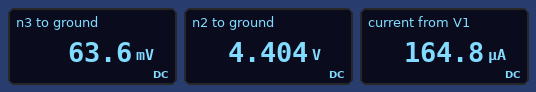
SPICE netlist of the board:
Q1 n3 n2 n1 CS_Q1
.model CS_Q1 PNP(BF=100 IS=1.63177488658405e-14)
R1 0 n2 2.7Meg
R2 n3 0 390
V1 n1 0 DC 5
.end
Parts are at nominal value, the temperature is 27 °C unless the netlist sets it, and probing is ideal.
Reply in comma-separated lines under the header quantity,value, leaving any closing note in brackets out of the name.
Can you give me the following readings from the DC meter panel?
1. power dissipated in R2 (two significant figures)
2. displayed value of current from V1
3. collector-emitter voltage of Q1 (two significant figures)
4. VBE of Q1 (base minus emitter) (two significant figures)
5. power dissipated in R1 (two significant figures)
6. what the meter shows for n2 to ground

quantity,value
power dissipated in R2,10 µW
displayed value of current from V1,164.8 µA
collector-emitter voltage of Q1,-4.9 V
VBE of Q1 (base minus emitter),-600 mV
power dissipated in R1,7.2 µW
what the meter shows for n2 to ground,4.404 V
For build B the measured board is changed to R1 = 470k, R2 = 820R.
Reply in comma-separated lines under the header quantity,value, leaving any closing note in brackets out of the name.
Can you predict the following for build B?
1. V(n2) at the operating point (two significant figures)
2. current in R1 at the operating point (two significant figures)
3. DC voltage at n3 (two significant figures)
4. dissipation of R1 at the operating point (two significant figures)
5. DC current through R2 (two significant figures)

quantity,value
V(n2) at the operating point,4.4 V
current in R1 at the operating point,9.3 µA
DC voltage at n3,760 mV
dissipation of R1 at the operating point,40 µW
DC current through R2,930 µA
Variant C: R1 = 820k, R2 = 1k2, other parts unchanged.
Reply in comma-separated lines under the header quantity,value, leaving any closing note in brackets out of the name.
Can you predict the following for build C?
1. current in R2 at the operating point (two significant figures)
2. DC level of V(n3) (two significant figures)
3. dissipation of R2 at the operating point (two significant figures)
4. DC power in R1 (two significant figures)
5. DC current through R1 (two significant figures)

quantity,value
current in R2 at the operating point,530 µA
DC level of V(n3),640 mV
dissipation of R2 at the operating point,340 µW
DC power in R1,23 µW
DC current through R1,5.3 µA
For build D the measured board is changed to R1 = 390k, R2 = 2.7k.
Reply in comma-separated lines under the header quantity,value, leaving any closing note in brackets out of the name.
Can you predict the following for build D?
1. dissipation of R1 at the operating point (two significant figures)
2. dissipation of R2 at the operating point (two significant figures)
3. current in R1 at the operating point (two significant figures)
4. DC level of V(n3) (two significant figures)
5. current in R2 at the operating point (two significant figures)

quantity,value
dissipation of R1 at the operating point,49 µW
dissipation of R2 at the operating point,3.4 mW
current in R1 at the operating point,11 µA
DC level of V(n3),3.0 V
current in R2 at the operating point,1.1 mA
